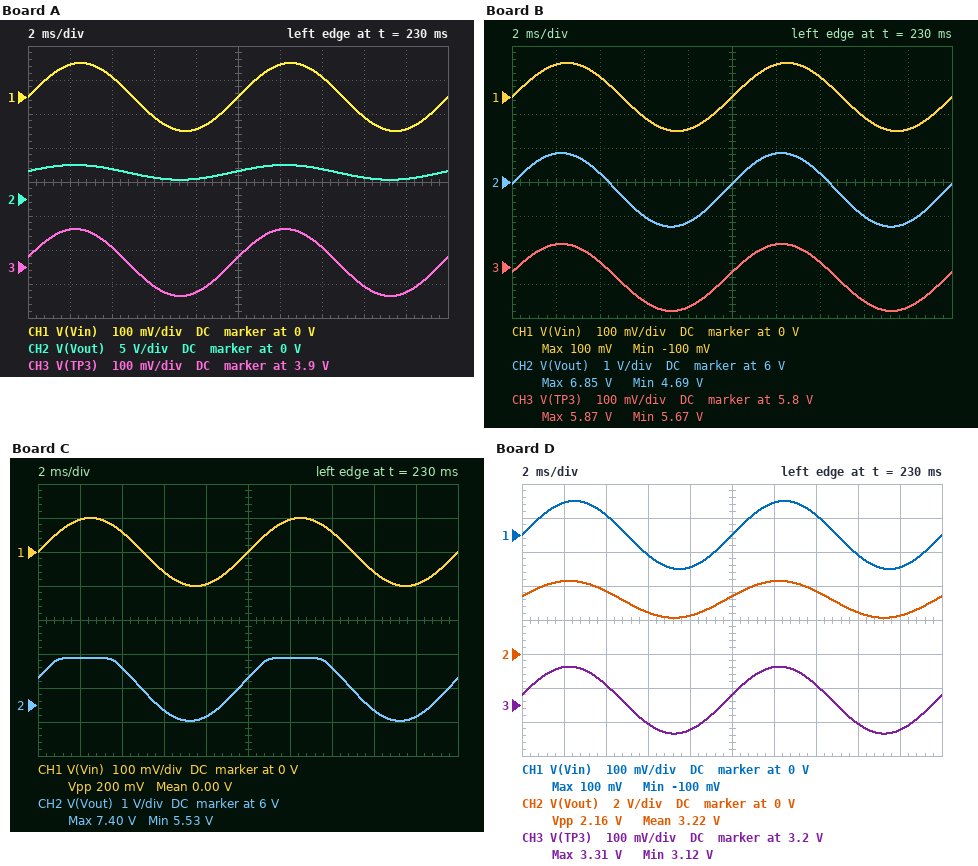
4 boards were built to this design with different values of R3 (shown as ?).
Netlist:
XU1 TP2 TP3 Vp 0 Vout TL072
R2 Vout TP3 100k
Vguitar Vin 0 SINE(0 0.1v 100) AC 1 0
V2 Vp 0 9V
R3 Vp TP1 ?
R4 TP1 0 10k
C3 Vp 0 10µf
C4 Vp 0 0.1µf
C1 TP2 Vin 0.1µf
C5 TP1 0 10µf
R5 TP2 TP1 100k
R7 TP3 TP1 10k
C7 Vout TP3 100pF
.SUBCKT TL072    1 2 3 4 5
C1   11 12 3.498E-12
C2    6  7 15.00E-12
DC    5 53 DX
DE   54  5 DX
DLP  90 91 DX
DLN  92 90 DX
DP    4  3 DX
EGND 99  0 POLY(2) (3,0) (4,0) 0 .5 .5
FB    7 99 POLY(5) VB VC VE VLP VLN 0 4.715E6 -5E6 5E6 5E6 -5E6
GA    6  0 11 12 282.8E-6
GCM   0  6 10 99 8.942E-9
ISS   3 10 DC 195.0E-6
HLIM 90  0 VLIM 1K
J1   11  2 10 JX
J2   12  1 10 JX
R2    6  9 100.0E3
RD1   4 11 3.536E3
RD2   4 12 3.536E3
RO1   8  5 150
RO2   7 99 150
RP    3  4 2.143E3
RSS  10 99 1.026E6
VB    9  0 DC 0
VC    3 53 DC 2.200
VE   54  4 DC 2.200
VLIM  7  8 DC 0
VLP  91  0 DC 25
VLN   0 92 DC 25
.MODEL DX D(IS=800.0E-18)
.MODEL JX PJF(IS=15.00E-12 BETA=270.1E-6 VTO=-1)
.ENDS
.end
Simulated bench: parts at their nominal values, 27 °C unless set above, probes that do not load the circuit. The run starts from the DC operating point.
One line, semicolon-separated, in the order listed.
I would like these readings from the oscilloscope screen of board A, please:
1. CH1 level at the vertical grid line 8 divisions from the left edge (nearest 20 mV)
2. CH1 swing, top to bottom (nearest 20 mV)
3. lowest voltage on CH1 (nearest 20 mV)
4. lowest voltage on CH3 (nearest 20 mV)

-60 mV; 200 mV; -100 mV; 3.82 V
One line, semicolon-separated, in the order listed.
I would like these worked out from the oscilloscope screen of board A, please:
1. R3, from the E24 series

13 kΩ
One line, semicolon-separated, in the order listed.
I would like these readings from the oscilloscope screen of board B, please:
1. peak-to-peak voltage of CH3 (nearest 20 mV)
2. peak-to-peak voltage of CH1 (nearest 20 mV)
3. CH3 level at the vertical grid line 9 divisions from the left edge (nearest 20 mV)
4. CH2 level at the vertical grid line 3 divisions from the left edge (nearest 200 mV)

200 mV; 200 mV; 5.68 V; 5.0 V
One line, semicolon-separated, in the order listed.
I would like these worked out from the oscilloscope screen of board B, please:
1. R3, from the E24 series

5.6 kΩ
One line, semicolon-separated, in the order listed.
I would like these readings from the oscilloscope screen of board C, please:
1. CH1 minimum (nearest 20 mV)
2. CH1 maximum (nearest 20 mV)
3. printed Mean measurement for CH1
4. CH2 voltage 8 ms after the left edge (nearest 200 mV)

-100 mV; 100 mV; 0.00 V; 5.6 V
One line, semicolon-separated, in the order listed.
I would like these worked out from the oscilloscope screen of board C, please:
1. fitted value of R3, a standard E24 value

3.6 kΩ
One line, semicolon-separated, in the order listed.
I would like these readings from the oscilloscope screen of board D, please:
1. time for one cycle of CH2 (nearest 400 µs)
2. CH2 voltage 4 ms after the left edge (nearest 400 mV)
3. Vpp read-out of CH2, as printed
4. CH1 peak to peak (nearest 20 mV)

10.0 ms; 3.6 V; 2.16 V; 200 mV
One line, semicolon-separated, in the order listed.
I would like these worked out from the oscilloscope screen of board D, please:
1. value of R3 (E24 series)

18 kΩ
